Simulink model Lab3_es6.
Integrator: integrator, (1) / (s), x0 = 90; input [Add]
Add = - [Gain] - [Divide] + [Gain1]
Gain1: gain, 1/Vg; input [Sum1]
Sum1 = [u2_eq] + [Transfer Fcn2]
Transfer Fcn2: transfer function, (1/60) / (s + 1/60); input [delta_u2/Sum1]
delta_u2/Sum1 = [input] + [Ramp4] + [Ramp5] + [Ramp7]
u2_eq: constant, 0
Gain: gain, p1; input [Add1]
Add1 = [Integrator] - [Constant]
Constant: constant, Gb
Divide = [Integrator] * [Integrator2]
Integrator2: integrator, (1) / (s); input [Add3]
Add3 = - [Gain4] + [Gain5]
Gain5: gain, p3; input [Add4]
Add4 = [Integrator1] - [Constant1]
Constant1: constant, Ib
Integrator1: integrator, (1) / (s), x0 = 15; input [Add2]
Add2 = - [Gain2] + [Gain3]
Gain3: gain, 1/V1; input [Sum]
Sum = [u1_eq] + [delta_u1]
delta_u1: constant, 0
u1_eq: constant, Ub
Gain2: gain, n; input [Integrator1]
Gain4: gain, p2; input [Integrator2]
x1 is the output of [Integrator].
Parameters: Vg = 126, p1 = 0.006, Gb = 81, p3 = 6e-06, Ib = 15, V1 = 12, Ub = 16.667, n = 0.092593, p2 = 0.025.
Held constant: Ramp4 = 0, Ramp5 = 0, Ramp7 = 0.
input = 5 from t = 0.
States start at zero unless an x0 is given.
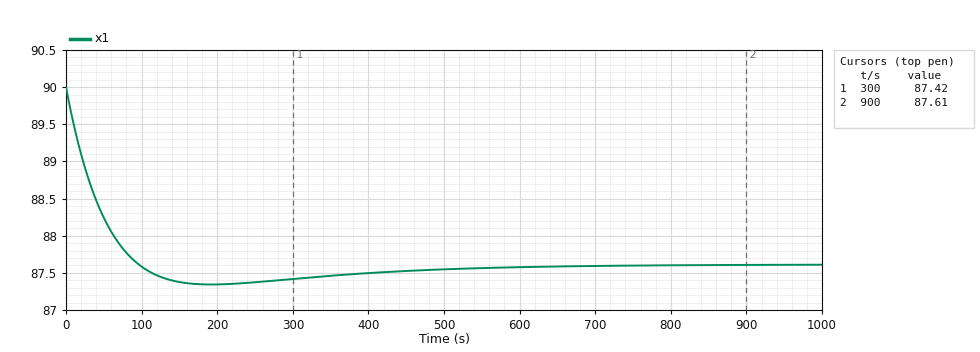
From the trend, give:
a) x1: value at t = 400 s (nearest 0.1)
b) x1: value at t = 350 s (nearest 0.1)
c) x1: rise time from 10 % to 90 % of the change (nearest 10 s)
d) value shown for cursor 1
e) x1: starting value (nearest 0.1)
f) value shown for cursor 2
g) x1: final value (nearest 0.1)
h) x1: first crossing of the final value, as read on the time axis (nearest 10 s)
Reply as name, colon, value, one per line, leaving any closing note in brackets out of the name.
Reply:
x1: value at t = 400 s: 87.5
x1: value at t = 350 s: 87.5
x1: rise time from 10 % to 90 % of the change: 70 s
value shown for cursor 1: 87.42
x1: starting value: 90.0
value shown for cursor 2: 87.61
x1: final value: 87.6
x1: first crossing of the final value, as read on the time axis: 100 s
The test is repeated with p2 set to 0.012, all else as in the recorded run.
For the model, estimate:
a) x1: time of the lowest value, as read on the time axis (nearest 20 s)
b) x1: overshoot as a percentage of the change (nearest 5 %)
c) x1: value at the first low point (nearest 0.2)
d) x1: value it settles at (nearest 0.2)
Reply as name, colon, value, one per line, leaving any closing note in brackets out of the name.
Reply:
x1: time of the lowest value, as read on the time axis: 200 s
x1: overshoot as a percentage of the change: 10 %
x1: value at the first low point: 87.4
x1: value it settles at: 87.6
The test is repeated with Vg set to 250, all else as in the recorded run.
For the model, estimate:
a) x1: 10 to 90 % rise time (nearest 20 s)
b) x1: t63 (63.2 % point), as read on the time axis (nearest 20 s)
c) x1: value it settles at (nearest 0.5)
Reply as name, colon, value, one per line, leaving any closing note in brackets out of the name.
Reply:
x1: 10 to 90 % rise time: 300 s
x1: t63 (63.2 % point), as read on the time axis: 120 s
x1: value it settles at: 84.5
